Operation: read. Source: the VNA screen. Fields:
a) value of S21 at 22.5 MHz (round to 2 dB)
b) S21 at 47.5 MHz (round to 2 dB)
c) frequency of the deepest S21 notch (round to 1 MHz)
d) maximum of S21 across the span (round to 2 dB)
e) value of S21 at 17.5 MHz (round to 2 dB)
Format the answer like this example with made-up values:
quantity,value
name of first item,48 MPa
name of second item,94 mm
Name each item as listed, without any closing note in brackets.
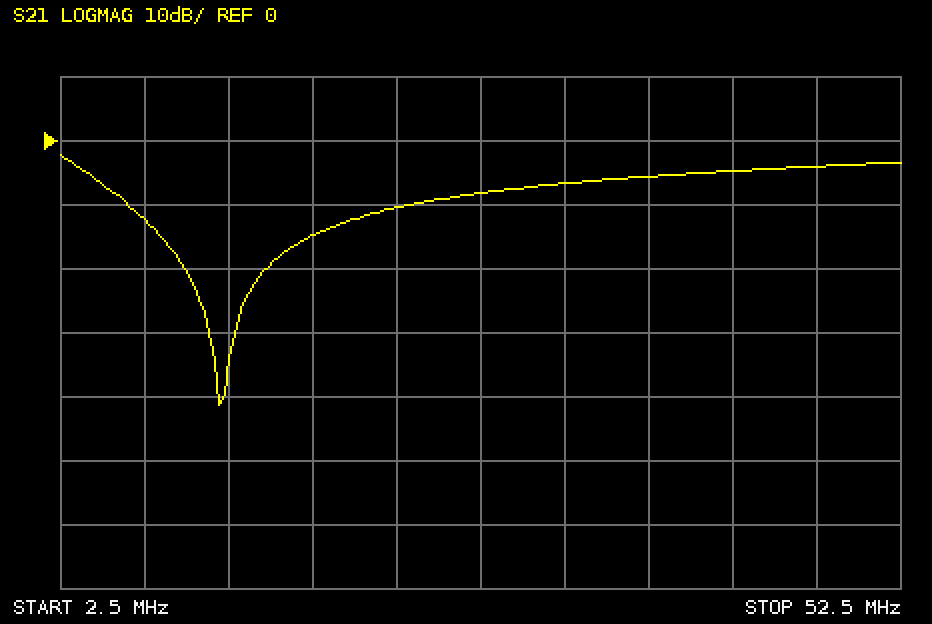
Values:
quantity,value
value of S21 at 22.5 MHz,-10 dB
S21 at 47.5 MHz,-4 dB
frequency of the deepest S21 notch,12 MHz
maximum of S21 across the span,-2 dB
value of S21 at 17.5 MHz,-14 dB
